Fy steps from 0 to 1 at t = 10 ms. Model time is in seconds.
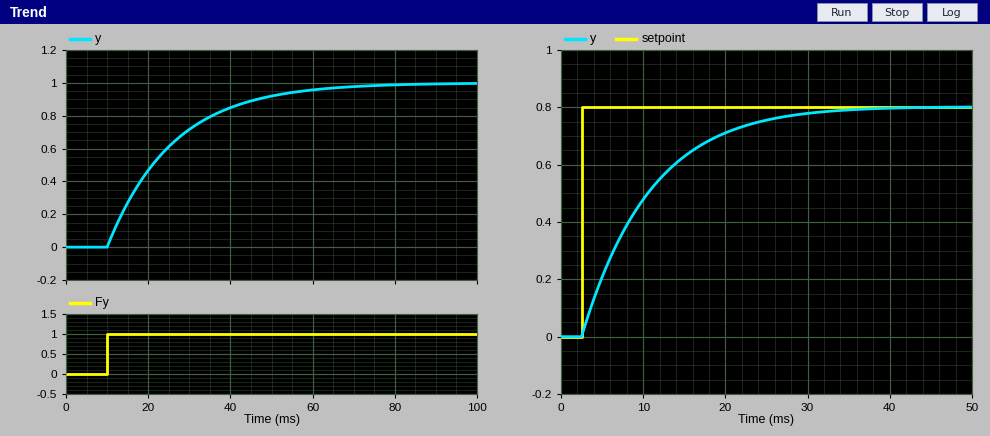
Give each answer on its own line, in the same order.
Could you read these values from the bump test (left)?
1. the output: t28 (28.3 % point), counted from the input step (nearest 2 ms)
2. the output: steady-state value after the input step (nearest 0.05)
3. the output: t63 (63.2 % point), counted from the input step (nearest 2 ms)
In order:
6 ms
1.00
16 ms
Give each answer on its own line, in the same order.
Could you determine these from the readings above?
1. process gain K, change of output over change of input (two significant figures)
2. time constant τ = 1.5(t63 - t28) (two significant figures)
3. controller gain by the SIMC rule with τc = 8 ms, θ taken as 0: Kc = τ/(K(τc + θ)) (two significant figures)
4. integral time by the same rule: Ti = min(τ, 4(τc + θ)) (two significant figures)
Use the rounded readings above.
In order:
1.0
15 ms
1.9
15 ms
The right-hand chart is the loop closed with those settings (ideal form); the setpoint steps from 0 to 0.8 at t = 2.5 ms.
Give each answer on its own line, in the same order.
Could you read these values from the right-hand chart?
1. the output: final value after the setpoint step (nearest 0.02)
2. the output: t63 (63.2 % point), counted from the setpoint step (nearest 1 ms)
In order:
0.80
8 ms
